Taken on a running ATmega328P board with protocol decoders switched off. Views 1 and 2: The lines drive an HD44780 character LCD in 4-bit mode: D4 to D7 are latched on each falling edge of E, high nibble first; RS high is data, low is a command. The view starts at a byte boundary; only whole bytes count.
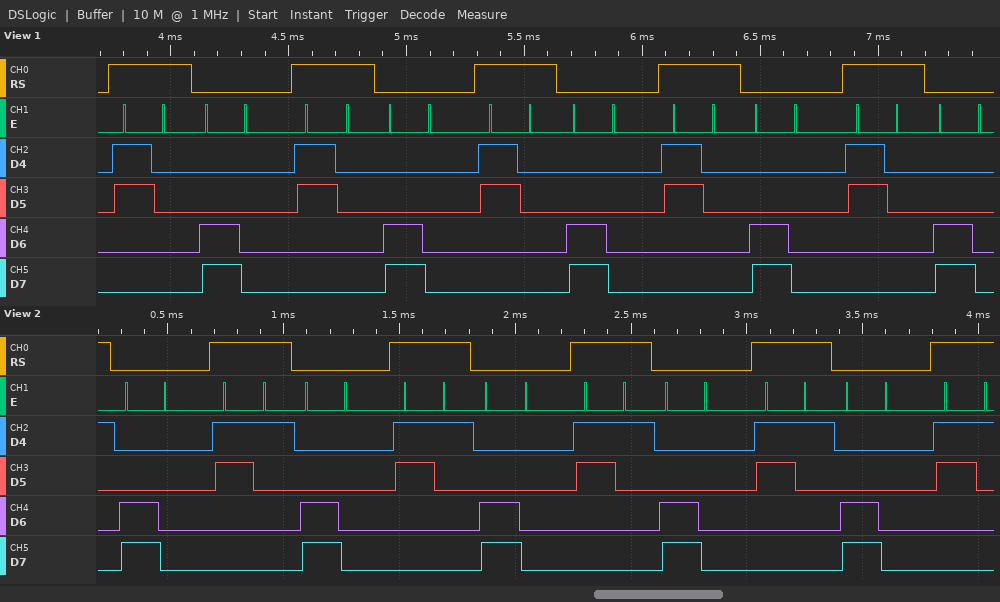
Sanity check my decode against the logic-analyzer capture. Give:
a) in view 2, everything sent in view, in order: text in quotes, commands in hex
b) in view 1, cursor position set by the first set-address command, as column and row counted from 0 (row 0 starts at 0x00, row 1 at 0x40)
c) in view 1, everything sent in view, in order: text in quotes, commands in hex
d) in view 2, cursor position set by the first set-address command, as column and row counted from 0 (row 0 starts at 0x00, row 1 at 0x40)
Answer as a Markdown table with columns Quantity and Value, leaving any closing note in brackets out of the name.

| Quantity | Value |
|---|---|
| in view 2, everything sent in view, in order: text in quotes, commands in hex | 0xC0 "1" 0xC0 "1" 0xC0 "1" 0xC0 "1" 0xC0 "1" |
| in view 1, cursor position set by the first set-address command, as column and row counted from 0 | column 0, row 1 |
| in view 1, everything sent in view, in order: text in quotes, commands in hex | "0" 0xC0 "0" 0xC0 "0" 0xC0 "0" 0xC0 "0" 0xC0 |
| in view 2, cursor position set by the first set-address command, as column and row counted from 0 | column 0, row 1 |
